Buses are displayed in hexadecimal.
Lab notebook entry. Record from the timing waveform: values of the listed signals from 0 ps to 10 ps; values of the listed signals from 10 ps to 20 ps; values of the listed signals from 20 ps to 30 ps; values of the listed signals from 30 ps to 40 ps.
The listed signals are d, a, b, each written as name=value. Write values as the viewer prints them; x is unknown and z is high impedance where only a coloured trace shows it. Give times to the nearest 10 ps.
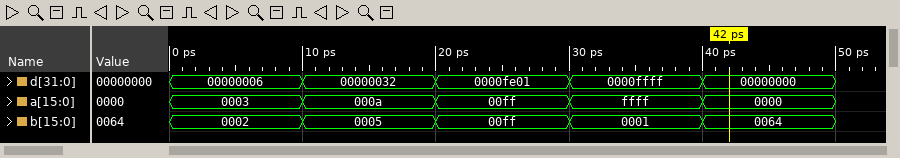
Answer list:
d=00000006, a=0003, b=0002
d=00000032, a=000a, b=0005
d=0000fe01, a=00ff, b=00ff
d=0000ffff, a=ffff, b=0001
